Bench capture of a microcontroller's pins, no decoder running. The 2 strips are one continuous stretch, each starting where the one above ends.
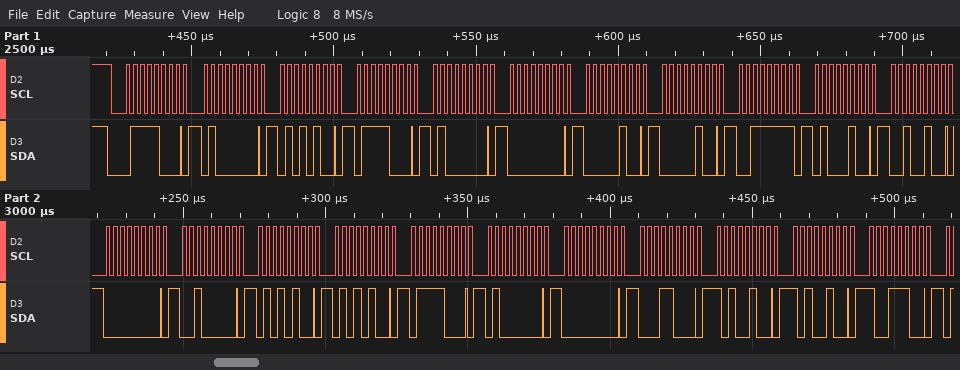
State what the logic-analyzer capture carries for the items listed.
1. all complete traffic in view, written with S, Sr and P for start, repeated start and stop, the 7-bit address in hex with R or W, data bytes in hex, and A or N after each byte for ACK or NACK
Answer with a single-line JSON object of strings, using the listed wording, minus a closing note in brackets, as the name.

{"all complete traffic in view, written with S, Sr and P for start, repeated start and stop, the 7-bit address in hex with R or W, data bytes in hex, and A or N after each byte for ACK or NACK": "S 3CW A 40 A 54 A 78 A 40 A 00 A 04 A 04 A 3F A 44 A 24 A 00 A 20 A 54 A 54 A 78 A 40 A 00 A 18 A A4 A A4 A 9C A"}
